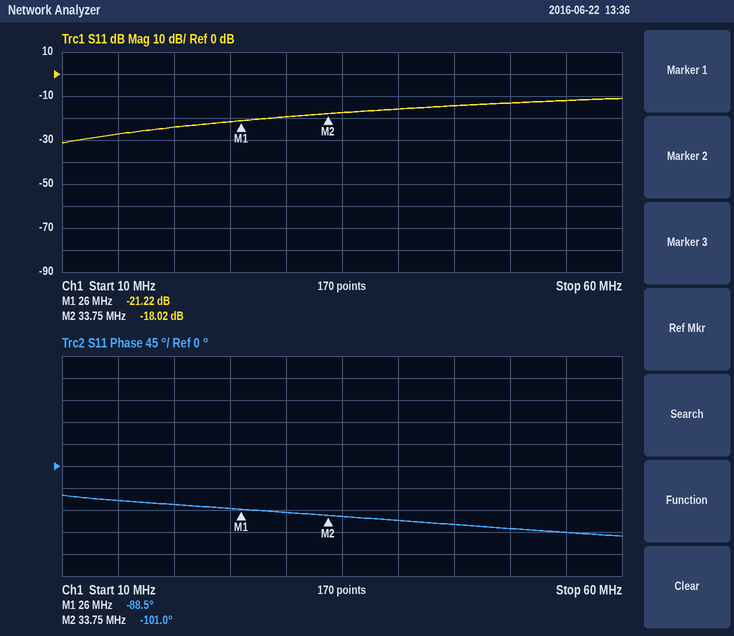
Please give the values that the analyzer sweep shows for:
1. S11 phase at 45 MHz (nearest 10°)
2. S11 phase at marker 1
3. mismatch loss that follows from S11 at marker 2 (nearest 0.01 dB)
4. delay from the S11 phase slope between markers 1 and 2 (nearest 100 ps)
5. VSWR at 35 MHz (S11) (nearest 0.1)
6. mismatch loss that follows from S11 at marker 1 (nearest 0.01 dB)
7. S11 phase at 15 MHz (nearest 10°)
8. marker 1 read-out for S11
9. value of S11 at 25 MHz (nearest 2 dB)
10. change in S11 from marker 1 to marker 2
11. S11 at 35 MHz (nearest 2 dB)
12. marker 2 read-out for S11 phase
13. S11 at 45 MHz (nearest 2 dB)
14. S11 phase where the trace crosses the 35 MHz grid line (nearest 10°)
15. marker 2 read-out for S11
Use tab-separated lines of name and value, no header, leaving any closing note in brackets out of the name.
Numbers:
S11 phase at 45 MHz	-120°
S11 phase at marker 1	-88.5°
mismatch loss that follows from S11 at marker 2	0.07 dB
delay from the S11 phase slope between markers 1 and 2	4.5 ns
VSWR at 35 MHz (S11)	1.3
mismatch loss that follows from S11 at marker 1	0.03 dB
S11 phase at 15 MHz	-70°
marker 1 read-out for S11	-21.22 dB
value of S11 at 25 MHz	-22 dB
change in S11 from marker 1 to marker 2	3.20 dB
S11 at 35 MHz	-18 dB
marker 2 read-out for S11 phase	-101.0°
S11 at 45 MHz	-14 dB
S11 phase where the trace crosses the 35 MHz grid line	-100°
marker 2 read-out for S11	-18.02 dB
